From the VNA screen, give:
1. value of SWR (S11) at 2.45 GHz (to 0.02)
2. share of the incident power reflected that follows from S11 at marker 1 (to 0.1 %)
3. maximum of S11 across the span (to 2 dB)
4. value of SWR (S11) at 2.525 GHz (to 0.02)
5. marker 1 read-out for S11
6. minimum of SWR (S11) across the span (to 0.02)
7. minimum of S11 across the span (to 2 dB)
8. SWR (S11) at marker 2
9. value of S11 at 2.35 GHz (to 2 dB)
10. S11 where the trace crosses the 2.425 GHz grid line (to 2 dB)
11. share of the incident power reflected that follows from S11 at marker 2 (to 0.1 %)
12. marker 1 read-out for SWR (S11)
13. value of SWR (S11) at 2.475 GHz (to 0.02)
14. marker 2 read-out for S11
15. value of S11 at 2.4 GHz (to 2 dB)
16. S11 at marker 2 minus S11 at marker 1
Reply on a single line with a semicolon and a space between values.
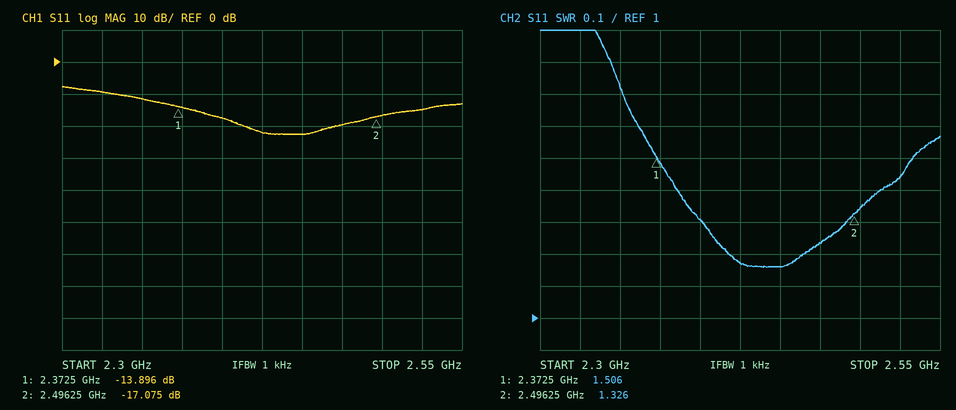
1.16; 4.1 %; -8 dB; 1.44; -13.896 dB; 1.16; -22 dB; 1.326; -12 dB; -22 dB; 2.0 %; 1.506; 1.24; -17.075 dB; -18 dB; -3.179 dB
